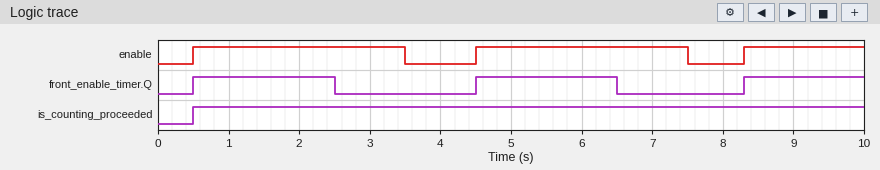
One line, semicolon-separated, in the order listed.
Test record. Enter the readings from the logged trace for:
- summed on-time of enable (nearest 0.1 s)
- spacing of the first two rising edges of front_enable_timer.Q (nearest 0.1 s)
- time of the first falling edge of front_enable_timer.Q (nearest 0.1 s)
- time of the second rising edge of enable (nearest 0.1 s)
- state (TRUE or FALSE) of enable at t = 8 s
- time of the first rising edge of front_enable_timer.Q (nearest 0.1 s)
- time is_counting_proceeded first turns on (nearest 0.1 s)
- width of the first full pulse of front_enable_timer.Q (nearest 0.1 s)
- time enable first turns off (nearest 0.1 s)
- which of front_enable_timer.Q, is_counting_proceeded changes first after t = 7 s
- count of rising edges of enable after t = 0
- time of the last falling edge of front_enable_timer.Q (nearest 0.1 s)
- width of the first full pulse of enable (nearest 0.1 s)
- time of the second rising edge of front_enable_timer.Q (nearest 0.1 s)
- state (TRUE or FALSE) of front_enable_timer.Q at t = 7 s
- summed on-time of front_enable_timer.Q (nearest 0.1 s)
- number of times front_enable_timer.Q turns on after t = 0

7.7 s; 4.0 s; 2.5 s; 4.5 s; FALSE; 0.5 s; 0.5 s; 2.0 s; 3.5 s; front_enable_timer.Q; 3; 6.5 s; 3.0 s; 4.5 s; FALSE; 5.7 s; 3
